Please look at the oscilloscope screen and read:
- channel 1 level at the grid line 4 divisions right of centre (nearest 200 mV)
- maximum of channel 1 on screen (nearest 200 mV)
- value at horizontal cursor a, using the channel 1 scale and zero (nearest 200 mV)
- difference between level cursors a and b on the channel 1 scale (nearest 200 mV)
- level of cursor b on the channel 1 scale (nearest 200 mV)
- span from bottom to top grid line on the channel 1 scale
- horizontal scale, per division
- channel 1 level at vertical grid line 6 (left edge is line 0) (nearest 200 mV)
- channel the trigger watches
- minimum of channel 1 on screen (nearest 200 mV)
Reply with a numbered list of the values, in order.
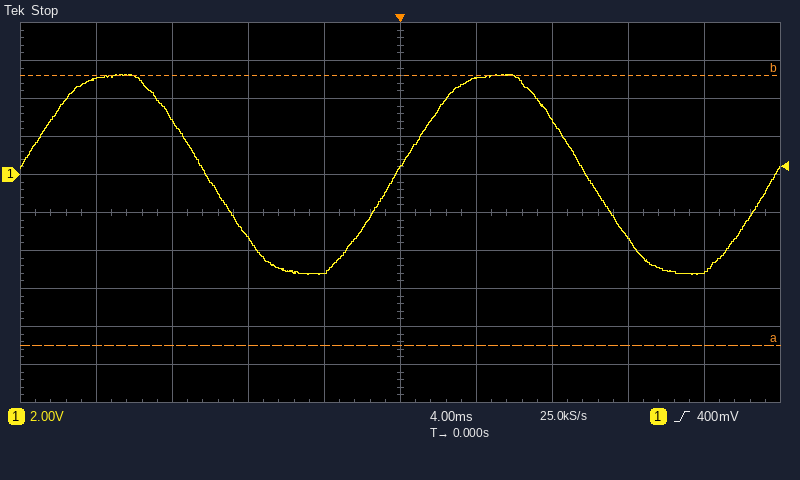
1. -5.0 V
2. 5.2 V
3. -9.0 V
4. 14.2 V
5. 5.2 V
6. 20 V
7. 4 ms
8. 5.0 V
9. channel 1
10. -5.2 V
